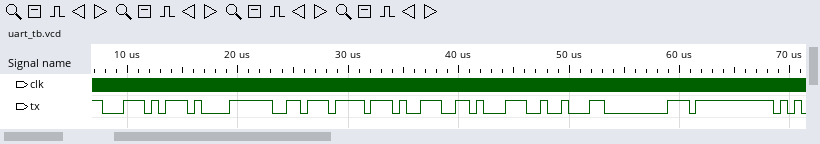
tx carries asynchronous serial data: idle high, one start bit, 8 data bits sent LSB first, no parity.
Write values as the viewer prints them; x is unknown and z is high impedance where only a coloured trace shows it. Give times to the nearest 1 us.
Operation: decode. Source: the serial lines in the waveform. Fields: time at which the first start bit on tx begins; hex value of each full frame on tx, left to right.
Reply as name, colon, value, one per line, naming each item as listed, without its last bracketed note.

time at which the first start bit on tx begins: 8 us
hex value of each full frame on tx, left to right: 5C, E1, 76, 97, 16, 12, 00, FF
